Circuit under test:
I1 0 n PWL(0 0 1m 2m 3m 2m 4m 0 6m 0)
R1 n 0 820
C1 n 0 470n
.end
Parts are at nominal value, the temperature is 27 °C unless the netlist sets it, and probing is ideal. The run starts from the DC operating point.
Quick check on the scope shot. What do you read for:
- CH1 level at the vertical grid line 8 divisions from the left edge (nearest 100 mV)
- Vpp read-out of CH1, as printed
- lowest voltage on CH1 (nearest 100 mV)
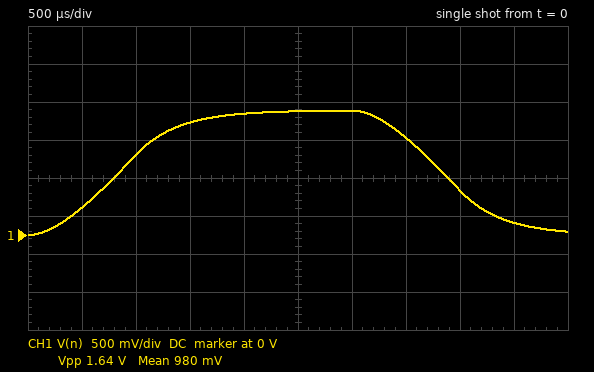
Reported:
600 mV
1.64 V
0 V
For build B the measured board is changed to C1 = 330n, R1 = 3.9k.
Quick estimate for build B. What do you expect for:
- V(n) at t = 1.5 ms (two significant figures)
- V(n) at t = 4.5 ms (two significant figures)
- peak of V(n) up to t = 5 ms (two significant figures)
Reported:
4.1 V
3.3 V
6.7 V
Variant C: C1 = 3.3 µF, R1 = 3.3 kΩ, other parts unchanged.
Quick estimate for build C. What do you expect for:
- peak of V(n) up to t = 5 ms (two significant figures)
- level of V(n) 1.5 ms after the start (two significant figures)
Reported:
1.5 V
580 mV
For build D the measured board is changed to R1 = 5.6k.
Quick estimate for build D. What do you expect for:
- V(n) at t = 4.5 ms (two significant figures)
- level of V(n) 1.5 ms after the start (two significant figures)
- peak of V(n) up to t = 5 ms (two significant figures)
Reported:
5.2 V
3.5 V
7.1 V
